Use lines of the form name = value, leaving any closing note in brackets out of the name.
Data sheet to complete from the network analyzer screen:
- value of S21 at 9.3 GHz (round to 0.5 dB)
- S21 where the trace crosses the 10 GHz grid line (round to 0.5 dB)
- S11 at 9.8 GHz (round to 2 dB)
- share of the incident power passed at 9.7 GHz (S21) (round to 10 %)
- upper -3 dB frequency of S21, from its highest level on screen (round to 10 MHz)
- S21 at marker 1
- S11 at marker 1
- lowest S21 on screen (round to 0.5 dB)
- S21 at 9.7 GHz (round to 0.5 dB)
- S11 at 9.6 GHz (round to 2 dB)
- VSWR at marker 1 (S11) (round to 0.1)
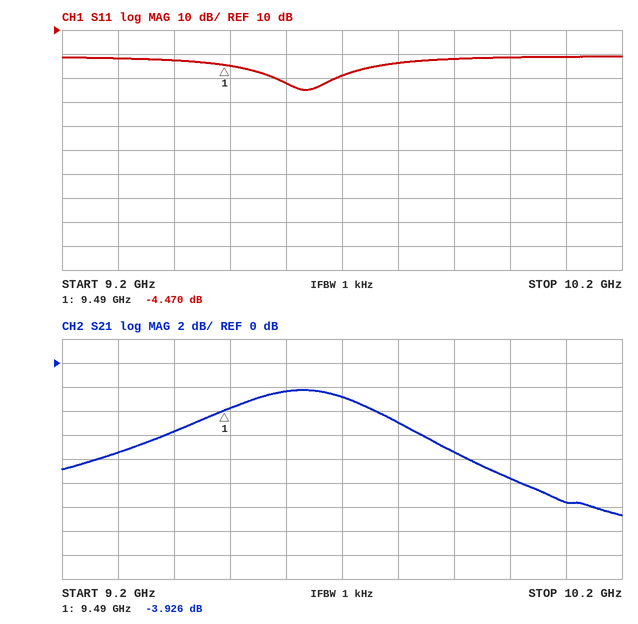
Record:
value of S21 at 9.3 GHz = -7.5 dB
S21 where the trace crosses the 10 GHz grid line = -9.5 dB
S11 at 9.8 GHz = -4 dB
share of the incident power passed at 9.7 GHz (S21) = 50 %
upper -3 dB frequency of S21, from its highest level on screen = 9.81 GHz
S21 at marker 1 = -3.926 dB
S11 at marker 1 = -4.470 dB
lowest S21 on screen = -12.5 dB
S21 at 9.7 GHz = -3.0 dB
S11 at 9.6 GHz = -12 dB
VSWR at marker 1 (S11) = 4.0
